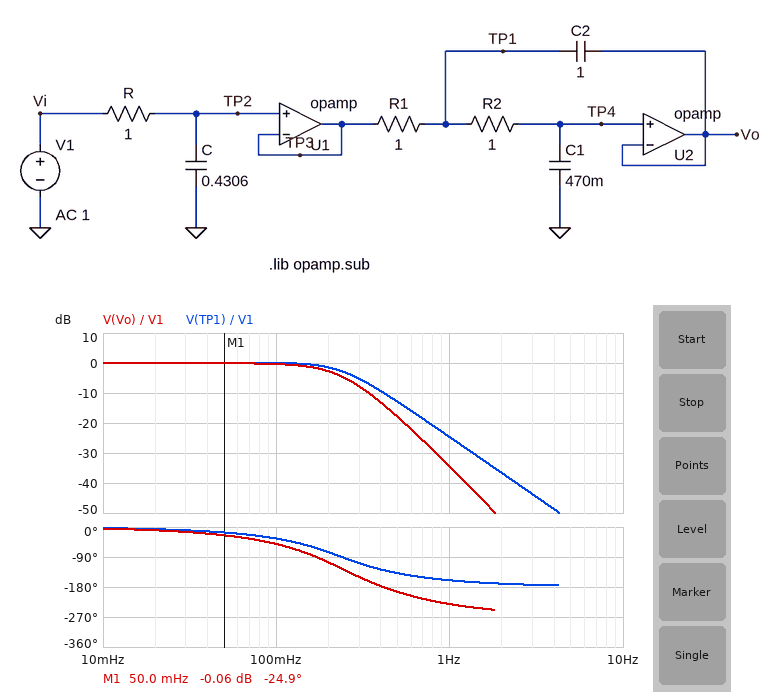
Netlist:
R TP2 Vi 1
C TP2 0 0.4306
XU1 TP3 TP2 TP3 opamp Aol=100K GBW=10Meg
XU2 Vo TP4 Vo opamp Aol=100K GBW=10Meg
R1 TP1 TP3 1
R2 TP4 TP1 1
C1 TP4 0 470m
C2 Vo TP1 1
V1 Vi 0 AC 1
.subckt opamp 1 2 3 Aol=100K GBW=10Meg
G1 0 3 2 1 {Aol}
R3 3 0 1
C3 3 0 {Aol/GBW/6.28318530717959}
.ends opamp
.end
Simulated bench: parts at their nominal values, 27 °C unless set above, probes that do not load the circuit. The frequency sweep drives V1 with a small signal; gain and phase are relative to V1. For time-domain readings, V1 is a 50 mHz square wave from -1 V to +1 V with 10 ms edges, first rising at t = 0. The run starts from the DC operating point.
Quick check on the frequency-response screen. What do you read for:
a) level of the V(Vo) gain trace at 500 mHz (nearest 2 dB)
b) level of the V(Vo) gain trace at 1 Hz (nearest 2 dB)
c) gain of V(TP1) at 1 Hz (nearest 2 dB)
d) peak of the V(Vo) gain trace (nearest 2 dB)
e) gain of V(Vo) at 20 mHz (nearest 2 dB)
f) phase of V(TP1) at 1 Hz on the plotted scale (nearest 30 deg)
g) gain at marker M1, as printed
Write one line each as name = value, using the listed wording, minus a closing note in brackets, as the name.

level of the V(Vo) gain trace at 500 mHz = -18 dB
level of the V(Vo) gain trace at 1 Hz = -34 dB
gain of V(TP1) at 1 Hz = -24 dB
peak of the V(Vo) gain trace = 0 dB
gain of V(Vo) at 20 mHz = 0 dB
phase of V(TP1) at 1 Hz on the plotted scale = -150 deg
gain at marker M1, as printed = -0.06 dB
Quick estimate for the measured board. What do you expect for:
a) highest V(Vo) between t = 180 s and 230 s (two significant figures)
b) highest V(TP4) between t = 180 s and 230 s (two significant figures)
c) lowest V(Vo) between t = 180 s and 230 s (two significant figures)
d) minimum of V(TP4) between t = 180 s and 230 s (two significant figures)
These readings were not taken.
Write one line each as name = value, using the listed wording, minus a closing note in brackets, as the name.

highest V(Vo) between t = 180 s and 230 s = 1.1 V
highest V(TP4) between t = 180 s and 230 s = 1.1 V
lowest V(Vo) between t = 180 s and 230 s = -1.1 V
minimum of V(TP4) between t = 180 s and 230 s = -1.1 V
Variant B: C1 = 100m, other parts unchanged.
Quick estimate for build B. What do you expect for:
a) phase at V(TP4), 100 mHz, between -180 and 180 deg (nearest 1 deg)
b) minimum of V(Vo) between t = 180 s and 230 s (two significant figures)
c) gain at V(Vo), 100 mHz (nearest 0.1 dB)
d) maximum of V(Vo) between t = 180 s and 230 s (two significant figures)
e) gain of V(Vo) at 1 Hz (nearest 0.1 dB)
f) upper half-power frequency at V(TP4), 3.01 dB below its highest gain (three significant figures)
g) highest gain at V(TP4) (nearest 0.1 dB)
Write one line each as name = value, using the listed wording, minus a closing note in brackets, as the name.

phase at V(TP4), 100 mHz, between -180 and 180 deg = -23 deg
minimum of V(Vo) between t = 180 s and 230 s = -1.3 V
gain at V(Vo), 100 mHz = 0 dB
maximum of V(Vo) between t = 180 s and 230 s = 1.3 V
gain of V(Vo) at 1 Hz = -19.3 dB
upper half-power frequency at V(TP4), 3.01 dB below its highest gain = 552 mHz
highest gain at V(TP4) = 0.7 dB
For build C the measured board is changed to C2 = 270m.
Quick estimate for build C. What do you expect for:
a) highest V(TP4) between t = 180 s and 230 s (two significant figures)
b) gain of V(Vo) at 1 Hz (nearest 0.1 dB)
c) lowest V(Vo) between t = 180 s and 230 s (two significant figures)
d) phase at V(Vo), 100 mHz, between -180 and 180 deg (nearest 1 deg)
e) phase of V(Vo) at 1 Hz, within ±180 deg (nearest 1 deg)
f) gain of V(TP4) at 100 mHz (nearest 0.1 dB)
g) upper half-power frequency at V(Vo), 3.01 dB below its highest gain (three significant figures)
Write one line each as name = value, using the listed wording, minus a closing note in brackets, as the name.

highest V(TP4) between t = 180 s and 230 s = 1.0 V
gain of V(Vo) at 1 Hz = -26.3 dB
lowest V(Vo) between t = 180 s and 230 s = -1.0 V
phase at V(Vo), 100 mHz, between -180 and 180 deg = -47 deg
phase of V(Vo) at 1 Hz, within ±180 deg = 166 deg
gain of V(TP4) at 100 mHz = -1.3 dB
upper half-power frequency at V(Vo), 3.01 dB below its highest gain = 163 mHz
